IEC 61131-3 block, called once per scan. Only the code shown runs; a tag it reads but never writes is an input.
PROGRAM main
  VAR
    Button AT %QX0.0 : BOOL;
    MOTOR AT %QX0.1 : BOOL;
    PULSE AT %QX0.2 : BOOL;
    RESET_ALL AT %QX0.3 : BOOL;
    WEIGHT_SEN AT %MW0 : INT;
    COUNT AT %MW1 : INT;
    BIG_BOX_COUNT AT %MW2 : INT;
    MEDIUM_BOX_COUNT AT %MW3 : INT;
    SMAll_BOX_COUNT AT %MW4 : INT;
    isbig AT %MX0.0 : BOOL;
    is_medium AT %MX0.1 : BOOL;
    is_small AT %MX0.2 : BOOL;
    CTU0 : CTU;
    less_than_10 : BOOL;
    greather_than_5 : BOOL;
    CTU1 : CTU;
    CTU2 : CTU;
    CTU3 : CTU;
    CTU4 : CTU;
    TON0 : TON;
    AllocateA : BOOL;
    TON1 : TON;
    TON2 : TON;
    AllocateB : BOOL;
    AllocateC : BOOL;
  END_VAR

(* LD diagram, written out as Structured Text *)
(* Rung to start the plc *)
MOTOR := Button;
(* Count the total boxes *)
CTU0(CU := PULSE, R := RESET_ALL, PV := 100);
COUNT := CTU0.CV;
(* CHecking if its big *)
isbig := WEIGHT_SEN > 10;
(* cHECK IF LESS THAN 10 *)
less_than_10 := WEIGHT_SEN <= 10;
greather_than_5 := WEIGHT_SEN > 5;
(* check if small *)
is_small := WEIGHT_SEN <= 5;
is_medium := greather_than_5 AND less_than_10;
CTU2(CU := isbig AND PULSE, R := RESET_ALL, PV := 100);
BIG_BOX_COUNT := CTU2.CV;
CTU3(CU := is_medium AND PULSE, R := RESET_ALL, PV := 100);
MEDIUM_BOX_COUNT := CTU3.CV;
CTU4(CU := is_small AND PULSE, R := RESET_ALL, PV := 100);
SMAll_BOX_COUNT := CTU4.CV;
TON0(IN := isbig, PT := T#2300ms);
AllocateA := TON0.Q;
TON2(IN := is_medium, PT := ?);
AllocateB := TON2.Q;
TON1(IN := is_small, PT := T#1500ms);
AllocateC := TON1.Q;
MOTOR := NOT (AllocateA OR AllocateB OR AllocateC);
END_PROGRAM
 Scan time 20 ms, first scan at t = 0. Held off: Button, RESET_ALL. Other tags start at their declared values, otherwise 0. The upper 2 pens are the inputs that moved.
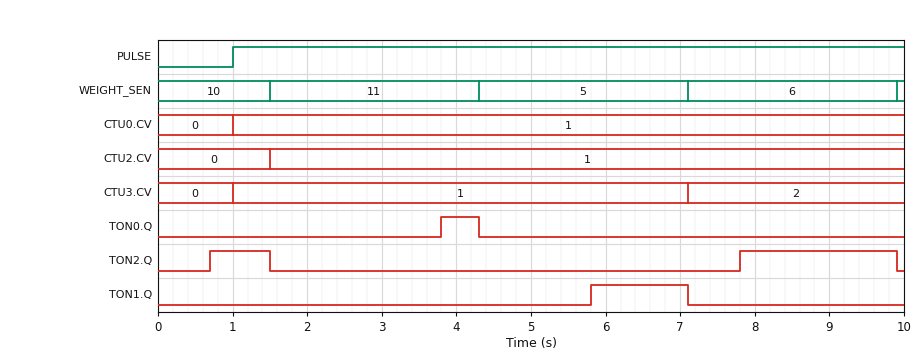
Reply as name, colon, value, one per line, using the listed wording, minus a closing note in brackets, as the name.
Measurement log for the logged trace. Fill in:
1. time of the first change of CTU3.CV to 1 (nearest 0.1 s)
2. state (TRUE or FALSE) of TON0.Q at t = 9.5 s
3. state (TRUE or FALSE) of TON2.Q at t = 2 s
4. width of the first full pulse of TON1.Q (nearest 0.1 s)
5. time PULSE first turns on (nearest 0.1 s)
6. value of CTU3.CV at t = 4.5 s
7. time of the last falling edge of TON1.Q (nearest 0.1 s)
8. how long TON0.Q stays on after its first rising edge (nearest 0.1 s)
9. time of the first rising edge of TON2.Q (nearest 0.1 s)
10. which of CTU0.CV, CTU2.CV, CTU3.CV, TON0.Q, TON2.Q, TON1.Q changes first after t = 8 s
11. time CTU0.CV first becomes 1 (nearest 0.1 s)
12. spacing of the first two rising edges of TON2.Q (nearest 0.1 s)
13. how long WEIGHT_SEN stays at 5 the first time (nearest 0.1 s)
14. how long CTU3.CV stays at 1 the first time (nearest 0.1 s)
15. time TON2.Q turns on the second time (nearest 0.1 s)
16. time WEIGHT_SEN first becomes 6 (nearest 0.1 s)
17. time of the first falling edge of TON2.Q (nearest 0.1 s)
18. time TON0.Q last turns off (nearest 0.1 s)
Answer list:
time of the first change of CTU3.CV to 1: 1.0 s
state (TRUE or FALSE) of TON0.Q at t = 9.5 s: FALSE
state (TRUE or FALSE) of TON2.Q at t = 2 s: FALSE
width of the first full pulse of TON1.Q: 1.3 s
time PULSE first turns on: 1.0 s
value of CTU3.CV at t = 4.5 s: 1
time of the last falling edge of TON1.Q: 7.1 s
how long TON0.Q stays on after its first rising edge: 0.5 s
time of the first rising edge of TON2.Q: 0.7 s
which of CTU0.CV, CTU2.CV, CTU3.CV, TON0.Q, TON2.Q, TON1.Q changes first after t = 8 s: TON2.Q
time CTU0.CV first becomes 1: 1.0 s
spacing of the first two rising edges of TON2.Q: 7.1 s
how long WEIGHT_SEN stays at 5 the first time: 2.8 s
how long CTU3.CV stays at 1 the first time: 6.1 s
time TON2.Q turns on the second time: 7.8 s
time WEIGHT_SEN first becomes 6: 7.1 s
time of the first falling edge of TON2.Q: 1.5 s
time TON0.Q last turns off: 4.3 s
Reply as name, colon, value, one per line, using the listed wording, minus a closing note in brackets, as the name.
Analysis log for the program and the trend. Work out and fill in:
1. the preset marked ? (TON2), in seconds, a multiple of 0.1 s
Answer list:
the preset marked ? (TON2), in seconds, a multiple of 0.1 s: 0.7 s
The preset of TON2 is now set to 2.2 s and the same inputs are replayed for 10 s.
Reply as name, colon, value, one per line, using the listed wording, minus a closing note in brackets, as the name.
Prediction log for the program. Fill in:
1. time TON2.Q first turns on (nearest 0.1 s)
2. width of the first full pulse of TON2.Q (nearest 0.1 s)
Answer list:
time TON2.Q first turns on: 9.3 s
width of the first full pulse of TON2.Q: 0.6 s
